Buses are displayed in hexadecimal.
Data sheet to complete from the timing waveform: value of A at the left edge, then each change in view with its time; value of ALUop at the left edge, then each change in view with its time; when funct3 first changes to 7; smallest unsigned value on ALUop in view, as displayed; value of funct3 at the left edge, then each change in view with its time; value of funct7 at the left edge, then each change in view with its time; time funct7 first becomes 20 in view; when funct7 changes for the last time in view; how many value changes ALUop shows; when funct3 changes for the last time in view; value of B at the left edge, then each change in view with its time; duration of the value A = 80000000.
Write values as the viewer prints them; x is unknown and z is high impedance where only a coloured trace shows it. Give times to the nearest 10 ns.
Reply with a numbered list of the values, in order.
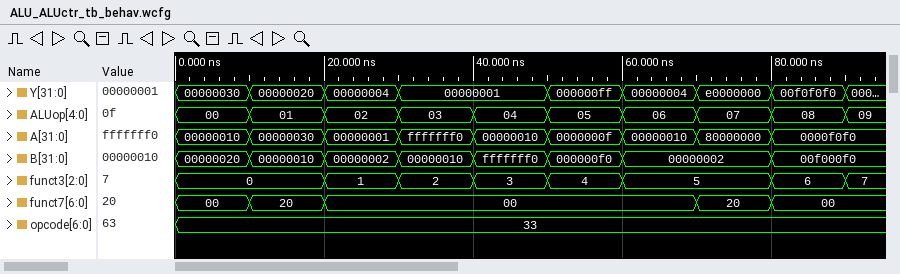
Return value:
1. 00000010, 00000030 at 10 ns, 00000001 at 20 ns, fffffff0 at 30 ns, 00000010 at 40 ns, 0000000f at 50 ns, 00000010 at 60 ns, 80000000 at 70 ns, 0000f0f0 at 80 ns
2. 00, 01 at 10 ns, 02 at 20 ns, 03 at 30 ns, 04 at 40 ns, 05 at 50 ns, 06 at 60 ns, 07 at 70 ns, 08 at 80 ns, 09 at 90 ns
3. 90 ns
4. 00
5. 0, 1 at 20 ns, 2 at 30 ns, 3 at 40 ns, 4 at 50 ns, 5 at 60 ns, 6 at 80 ns, 7 at 90 ns
6. 00, 20 at 10 ns, 00 at 20 ns, 20 at 70 ns, 00 at 80 ns
7. 10 ns
8. 80 ns
9. 9
10. 90 ns
11. 00000020, 00000010 at 10 ns, 00000002 at 20 ns, 00000010 at 30 ns, fffffff0 at 40 ns, 000000f0 at 50 ns, 00000002 at 60 ns, 00f000f0 at 80 ns
12. 10 ns
